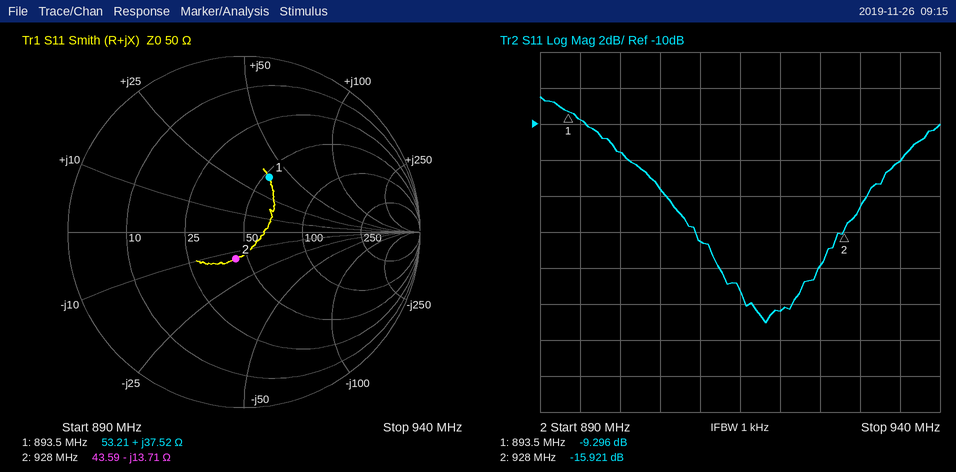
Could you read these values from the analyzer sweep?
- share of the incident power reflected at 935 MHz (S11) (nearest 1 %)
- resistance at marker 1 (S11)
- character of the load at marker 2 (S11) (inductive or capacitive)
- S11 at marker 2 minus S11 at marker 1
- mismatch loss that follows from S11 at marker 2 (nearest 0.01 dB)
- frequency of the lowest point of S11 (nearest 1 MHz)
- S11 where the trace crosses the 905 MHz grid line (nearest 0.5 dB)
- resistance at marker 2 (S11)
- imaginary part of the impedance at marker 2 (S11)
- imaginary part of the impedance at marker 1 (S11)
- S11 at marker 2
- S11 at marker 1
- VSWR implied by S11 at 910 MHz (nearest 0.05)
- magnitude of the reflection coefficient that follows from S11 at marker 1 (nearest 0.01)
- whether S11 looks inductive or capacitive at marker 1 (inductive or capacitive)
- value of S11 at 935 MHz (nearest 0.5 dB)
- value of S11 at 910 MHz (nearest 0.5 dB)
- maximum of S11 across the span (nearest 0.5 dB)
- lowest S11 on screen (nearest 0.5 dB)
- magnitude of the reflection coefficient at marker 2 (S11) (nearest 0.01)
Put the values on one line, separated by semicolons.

6 %; 53.21 Ω; capacitive; -6.625 dB; 0.11 dB; 918 MHz; -13.5 dB; 43.59 Ω; -13.71 Ω; +37.52 Ω; -15.921 dB; -9.296 dB; 1.35; 0.34; inductive; -12.0 dB; -16.5 dB; -8.5 dB; -21.0 dB; 0.16
